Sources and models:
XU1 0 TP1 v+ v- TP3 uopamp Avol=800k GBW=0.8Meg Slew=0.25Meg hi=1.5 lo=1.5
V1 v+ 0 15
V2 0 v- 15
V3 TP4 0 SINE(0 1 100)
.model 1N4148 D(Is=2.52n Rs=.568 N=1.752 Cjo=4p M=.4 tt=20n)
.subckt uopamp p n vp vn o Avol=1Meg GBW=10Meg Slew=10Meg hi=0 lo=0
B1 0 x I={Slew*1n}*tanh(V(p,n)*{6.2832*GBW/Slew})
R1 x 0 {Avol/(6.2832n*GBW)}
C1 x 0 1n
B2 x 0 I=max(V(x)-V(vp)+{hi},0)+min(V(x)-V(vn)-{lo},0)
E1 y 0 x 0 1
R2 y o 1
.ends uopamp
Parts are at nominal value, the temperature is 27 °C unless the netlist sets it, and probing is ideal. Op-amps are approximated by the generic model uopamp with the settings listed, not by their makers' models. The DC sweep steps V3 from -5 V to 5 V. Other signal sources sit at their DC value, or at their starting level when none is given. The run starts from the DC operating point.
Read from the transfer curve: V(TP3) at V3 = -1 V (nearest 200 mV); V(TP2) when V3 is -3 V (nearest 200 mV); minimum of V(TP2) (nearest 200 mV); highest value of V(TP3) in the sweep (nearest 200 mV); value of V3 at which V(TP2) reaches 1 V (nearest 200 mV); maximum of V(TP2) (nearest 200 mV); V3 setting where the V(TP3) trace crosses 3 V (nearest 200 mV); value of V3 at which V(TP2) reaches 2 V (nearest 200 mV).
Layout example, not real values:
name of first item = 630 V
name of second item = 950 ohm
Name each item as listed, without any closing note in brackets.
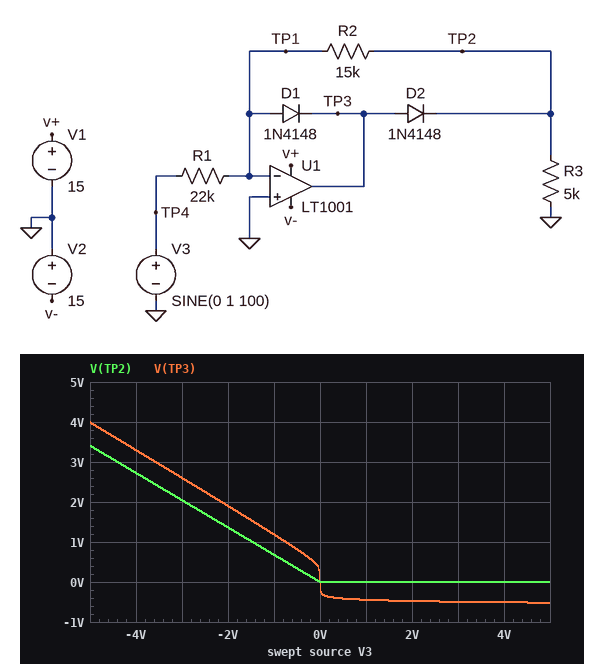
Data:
V(TP3) at V3 = -1 V = 1.2 V
V(TP2) when V3 is -3 V = 2.0 V
minimum of V(TP2) = 0 V
highest value of V(TP3) in the sweep = 4.0 V
value of V3 at which V(TP2) reaches 1 V = -1.4 V
maximum of V(TP2) = 3.4 V
V3 setting where the V(TP3) trace crosses 3 V = -3.6 V
value of V3 at which V(TP2) reaches 2 V = -3.0 V
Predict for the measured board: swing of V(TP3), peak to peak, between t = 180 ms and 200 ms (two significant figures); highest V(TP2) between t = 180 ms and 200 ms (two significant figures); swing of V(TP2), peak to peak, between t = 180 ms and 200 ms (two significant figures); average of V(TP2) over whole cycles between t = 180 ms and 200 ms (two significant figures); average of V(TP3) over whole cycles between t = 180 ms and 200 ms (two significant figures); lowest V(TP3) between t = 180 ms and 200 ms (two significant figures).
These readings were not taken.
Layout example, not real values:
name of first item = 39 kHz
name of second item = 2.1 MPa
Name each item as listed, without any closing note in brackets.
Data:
swing of V(TP3), peak to peak, between t = 180 ms and 200 ms = 1.6 V
highest V(TP2) between t = 180 ms and 200 ms = 680 mV
swing of V(TP2), peak to peak, between t = 180 ms and 200 ms = 680 mV
average of V(TP2) over whole cycles between t = 180 ms and 200 ms = 220 mV
average of V(TP3) over whole cycles between t = 180 ms and 200 ms = 250 mV
lowest V(TP3) between t = 180 ms and 200 ms = -440 mV
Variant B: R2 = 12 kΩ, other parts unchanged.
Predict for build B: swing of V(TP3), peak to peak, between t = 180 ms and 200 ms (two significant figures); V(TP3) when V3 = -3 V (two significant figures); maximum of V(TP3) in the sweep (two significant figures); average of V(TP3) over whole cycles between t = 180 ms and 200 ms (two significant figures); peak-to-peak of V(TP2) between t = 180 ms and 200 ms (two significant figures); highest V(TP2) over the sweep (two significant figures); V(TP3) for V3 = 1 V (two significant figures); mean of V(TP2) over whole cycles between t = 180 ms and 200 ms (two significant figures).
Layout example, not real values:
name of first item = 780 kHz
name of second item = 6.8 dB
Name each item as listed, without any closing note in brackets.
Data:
swing of V(TP3), peak to peak, between t = 180 ms and 200 ms = 1.5 V
V(TP3) when V3 = -3 V = 2.2 V
maximum of V(TP3) in the sweep = 3.3 V
average of V(TP3) over whole cycles between t = 180 ms and 200 ms = 200 mV
peak-to-peak of V(TP2) between t = 180 ms and 200 ms = 550 mV
highest V(TP2) over the sweep = 2.7 V
V(TP3) for V3 = 1 V = -440 mV
mean of V(TP2) over whole cycles between t = 180 ms and 200 ms = 170 mV
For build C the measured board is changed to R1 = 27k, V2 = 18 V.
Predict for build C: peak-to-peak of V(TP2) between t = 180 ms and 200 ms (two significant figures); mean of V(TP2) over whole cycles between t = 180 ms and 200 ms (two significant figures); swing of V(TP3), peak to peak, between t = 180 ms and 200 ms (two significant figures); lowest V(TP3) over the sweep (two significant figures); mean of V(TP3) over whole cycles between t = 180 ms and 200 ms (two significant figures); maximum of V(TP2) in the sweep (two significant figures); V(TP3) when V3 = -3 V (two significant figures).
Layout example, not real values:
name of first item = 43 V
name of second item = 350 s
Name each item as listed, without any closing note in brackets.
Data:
peak-to-peak of V(TP2) between t = 180 ms and 200 ms = 560 mV
mean of V(TP2) over whole cycles between t = 180 ms and 200 ms = 180 mV
swing of V(TP3), peak to peak, between t = 180 ms and 200 ms = 1.5 V
lowest V(TP3) over the sweep = -510 mV
mean of V(TP3) over whole cycles between t = 180 ms and 200 ms = 210 mV
maximum of V(TP2) in the sweep = 2.8 V
V(TP3) when V3 = -3 V = 2.2 V
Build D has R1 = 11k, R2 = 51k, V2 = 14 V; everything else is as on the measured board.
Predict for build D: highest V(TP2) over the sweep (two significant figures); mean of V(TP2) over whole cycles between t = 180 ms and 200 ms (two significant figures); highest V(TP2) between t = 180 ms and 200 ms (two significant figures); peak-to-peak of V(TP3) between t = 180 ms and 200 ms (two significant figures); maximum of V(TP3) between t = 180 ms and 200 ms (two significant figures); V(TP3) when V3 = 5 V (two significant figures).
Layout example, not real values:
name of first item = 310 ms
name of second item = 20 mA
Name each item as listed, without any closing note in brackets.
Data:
highest V(TP2) over the sweep = 13 V
mean of V(TP2) over whole cycles between t = 180 ms and 200 ms = 1.5 V
highest V(TP2) between t = 180 ms and 200 ms = 4.6 V
peak-to-peak of V(TP3) between t = 180 ms and 200 ms = 5.7 V
maximum of V(TP3) between t = 180 ms and 200 ms = 5.2 V
V(TP3) when V3 = 5 V = -550 mV
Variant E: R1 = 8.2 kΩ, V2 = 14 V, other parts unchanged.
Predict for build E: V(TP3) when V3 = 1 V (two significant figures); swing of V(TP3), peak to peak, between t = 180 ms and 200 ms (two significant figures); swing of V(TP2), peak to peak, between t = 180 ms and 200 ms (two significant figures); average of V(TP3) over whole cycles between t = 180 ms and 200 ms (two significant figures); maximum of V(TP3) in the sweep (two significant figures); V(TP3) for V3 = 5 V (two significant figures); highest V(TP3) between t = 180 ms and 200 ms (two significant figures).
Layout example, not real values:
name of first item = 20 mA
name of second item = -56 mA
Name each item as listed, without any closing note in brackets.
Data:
V(TP3) when V3 = 1 V = -490 mV
swing of V(TP3), peak to peak, between t = 180 ms and 200 ms = 2.9 V
swing of V(TP2), peak to peak, between t = 180 ms and 200 ms = 1.8 V
average of V(TP3) over whole cycles between t = 180 ms and 200 ms = 610 mV
maximum of V(TP3) in the sweep = 9.8 V
V(TP3) for V3 = 5 V = -560 mV
highest V(TP3) between t = 180 ms and 200 ms = 2.4 V
